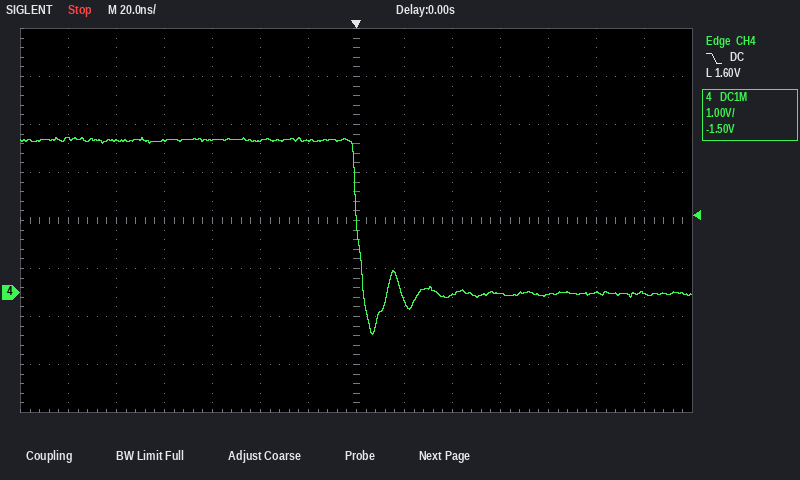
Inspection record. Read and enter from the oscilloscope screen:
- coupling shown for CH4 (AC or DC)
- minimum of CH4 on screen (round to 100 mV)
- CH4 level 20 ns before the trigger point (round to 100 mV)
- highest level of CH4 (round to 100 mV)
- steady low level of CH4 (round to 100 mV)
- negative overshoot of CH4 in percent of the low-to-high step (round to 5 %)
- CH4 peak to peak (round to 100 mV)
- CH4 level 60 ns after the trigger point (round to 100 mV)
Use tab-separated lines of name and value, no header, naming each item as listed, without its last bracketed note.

coupling shown for CH4	DC
minimum of CH4 on screen	-900 mV
CH4 level 20 ns before the trigger point	3.2 V
highest level of CH4	3.2 V
steady low level of CH4	0.0 V
negative overshoot of CH4 in percent of the low-to-high step	25 %
CH4 peak to peak	4.1 V
CH4 level 60 ns after the trigger point	0.0 V
